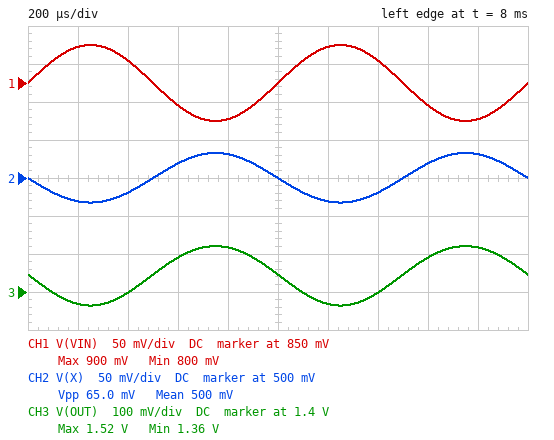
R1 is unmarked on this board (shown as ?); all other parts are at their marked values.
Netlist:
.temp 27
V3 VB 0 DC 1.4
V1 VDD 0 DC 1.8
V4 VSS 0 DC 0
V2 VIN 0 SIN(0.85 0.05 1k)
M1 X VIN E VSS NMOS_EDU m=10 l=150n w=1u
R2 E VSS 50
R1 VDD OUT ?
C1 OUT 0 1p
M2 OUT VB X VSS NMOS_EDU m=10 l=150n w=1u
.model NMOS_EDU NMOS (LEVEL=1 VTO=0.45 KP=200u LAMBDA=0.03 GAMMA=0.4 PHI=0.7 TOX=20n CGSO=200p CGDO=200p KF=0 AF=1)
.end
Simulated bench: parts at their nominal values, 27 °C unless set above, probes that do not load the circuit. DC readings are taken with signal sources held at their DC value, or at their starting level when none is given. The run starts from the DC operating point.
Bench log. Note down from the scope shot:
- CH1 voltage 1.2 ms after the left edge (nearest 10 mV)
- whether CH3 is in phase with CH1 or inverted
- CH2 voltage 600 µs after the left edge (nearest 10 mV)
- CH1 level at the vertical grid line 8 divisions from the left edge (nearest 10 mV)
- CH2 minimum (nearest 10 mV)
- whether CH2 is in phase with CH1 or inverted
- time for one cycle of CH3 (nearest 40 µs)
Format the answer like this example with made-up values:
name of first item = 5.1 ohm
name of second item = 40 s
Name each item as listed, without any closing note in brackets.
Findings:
CH1 voltage 1.2 ms after the left edge = 900 mV
whether CH3 is in phase with CH1 or inverted = inverted
CH2 voltage 600 µs after the left edge = 520 mV
CH1 level at the vertical grid line 8 divisions from the left edge = 820 mV
CH2 minimum = 470 mV
whether CH2 is in phase with CH1 or inverted = inverted
time for one cycle of CH3 = 1.00 ms
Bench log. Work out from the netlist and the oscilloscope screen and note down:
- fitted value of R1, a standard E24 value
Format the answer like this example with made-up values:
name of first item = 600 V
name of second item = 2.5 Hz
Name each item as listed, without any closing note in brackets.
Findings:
fitted value of R1, a standard E24 value = 430 Ω
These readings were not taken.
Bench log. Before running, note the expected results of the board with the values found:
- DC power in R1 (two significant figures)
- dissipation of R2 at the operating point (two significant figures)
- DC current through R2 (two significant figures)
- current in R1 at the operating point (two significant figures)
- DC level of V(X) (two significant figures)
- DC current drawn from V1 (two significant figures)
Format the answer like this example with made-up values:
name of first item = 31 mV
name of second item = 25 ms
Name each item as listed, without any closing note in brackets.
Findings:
DC power in R1 = 290 µW
dissipation of R2 at the operating point = 34 µW
DC current through R2 = 820 µA
current in R1 at the operating point = 820 µA
DC level of V(X) = 500 mV
DC current drawn from V1 = 820 µA
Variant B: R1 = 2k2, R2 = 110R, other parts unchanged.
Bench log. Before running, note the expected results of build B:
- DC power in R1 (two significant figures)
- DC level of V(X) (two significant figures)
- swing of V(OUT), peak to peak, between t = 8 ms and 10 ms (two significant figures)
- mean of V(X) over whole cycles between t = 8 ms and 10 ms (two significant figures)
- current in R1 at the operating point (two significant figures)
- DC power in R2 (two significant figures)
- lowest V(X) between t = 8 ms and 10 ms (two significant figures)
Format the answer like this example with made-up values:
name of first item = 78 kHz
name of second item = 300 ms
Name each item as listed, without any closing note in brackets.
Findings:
DC power in R1 = 880 µW
DC level of V(X) = 320 mV
swing of V(OUT), peak to peak, between t = 8 ms and 10 ms = 300 mV
mean of V(X) over whole cycles between t = 8 ms and 10 ms = 350 mV
current in R1 at the operating point = 630 µA
DC power in R2 = 44 µW
lowest V(X) between t = 8 ms and 10 ms = 260 mV
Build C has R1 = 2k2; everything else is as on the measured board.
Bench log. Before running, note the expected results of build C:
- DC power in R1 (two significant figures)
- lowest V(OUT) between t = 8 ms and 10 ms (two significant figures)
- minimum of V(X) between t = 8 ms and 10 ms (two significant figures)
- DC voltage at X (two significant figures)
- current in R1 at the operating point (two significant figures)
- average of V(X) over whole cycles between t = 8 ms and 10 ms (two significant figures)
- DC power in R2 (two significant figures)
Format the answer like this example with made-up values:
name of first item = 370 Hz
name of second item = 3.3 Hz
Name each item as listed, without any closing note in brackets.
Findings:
DC power in R1 = 1.0 mW
lowest V(OUT) between t = 8 ms and 10 ms = 270 mV
minimum of V(X) between t = 8 ms and 10 ms = 190 mV
DC voltage at X = 230 mV
current in R1 at the operating point = 680 µA
average of V(X) over whole cycles between t = 8 ms and 10 ms = 240 mV
DC power in R2 = 23 µW
